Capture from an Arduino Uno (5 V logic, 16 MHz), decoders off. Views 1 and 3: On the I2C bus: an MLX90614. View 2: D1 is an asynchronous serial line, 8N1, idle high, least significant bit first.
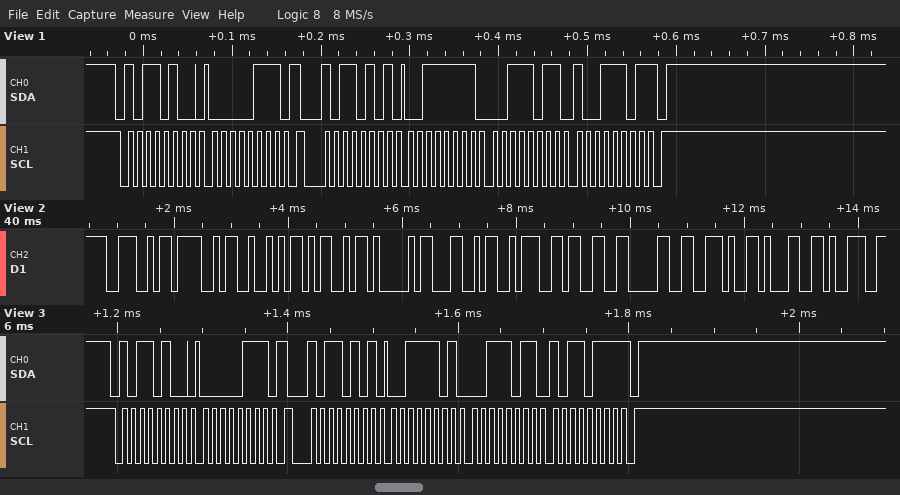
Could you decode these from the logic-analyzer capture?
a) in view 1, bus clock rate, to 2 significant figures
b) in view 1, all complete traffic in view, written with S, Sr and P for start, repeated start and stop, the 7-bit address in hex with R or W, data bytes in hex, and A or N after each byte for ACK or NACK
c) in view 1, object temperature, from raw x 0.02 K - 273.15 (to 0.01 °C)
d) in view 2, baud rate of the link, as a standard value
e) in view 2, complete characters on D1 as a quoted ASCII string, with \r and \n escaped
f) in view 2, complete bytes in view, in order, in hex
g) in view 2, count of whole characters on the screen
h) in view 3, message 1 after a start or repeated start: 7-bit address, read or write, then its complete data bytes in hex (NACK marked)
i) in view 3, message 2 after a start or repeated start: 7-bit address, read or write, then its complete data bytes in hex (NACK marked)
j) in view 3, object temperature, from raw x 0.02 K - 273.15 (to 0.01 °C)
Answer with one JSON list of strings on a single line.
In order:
["100 kHz", "S 5AW A 07 A Sr 5AR A 3F A 3B A 9D N P", "30.19 °C", "9600 baud", "\"NORMAL:30.19\"", "0x4E 0x4F 0x52 0x4D 0x41 0x4C 0x3A 0x33 0x30 0x2E 0x31 0x39", "12", "0x5A write: 07", "0x5A read: 3D 3B B7 NACK", "30.15 °C"]
